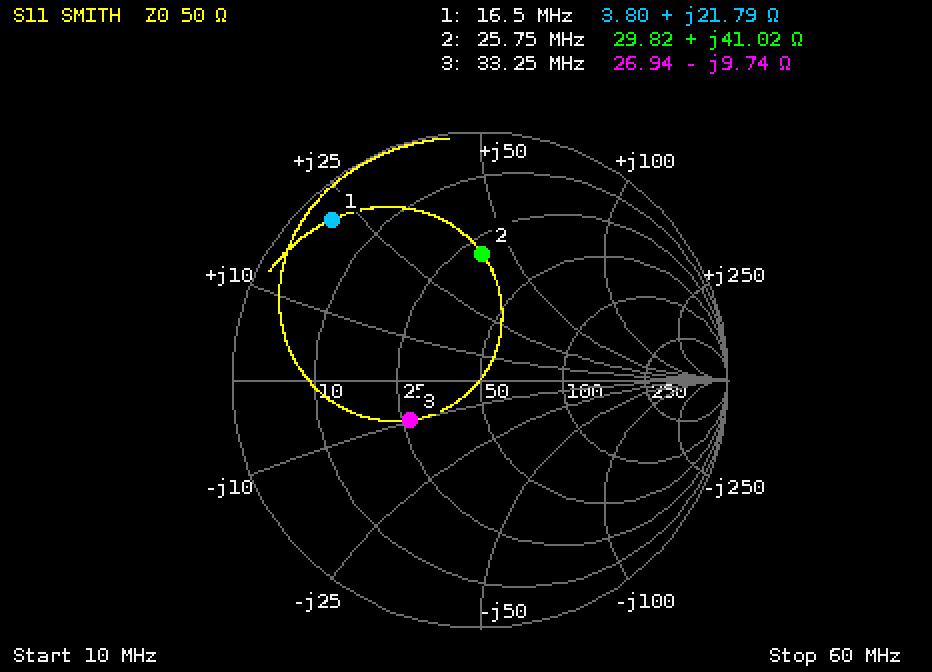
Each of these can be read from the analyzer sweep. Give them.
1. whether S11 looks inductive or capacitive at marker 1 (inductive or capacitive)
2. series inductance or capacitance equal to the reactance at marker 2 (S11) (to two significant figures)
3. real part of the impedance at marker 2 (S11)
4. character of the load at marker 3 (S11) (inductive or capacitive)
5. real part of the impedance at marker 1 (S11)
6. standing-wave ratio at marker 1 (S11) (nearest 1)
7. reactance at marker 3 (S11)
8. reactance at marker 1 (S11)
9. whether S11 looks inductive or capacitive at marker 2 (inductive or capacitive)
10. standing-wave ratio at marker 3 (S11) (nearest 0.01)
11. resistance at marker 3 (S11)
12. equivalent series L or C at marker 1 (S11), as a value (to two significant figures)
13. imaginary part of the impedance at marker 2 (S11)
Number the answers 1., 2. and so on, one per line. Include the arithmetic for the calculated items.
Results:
1. inductive
2. L = 41.02 Ω/(2π × 25.75 MHz) ≈ 254 nH, so 250 nH to two significant figures
3. 29.82 Ω
4. capacitive
5. 3.80 Ω
6. 16
7. -9.74 Ω
8. +21.79 Ω
9. inductive
10. 1.95
11. 26.94 Ω
12. L = 21.79 Ω/(2π × 16.5 MHz) ≈ 210 nH
13. +41.02 Ω
